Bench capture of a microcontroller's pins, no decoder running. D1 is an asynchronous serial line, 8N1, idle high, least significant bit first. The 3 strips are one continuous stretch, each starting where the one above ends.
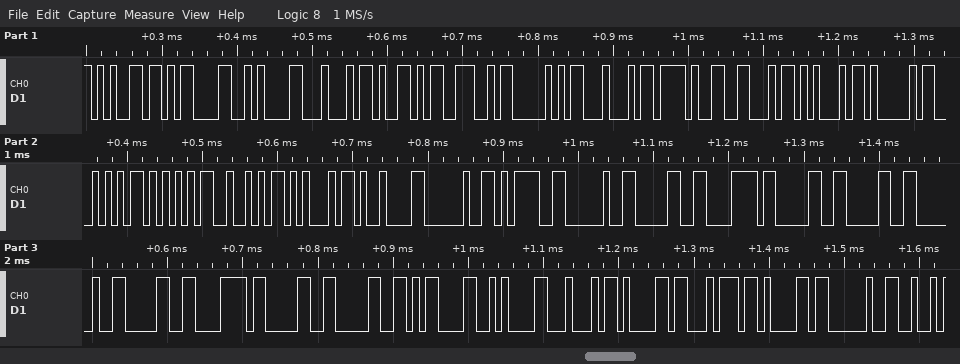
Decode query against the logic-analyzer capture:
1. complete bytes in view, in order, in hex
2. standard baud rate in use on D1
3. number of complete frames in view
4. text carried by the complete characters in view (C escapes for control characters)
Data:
65 0D 0A 44 59 4E 50 44 2F 46 45 41 54 55 52 45 09 20 3D 20 30 78 30 30 20 30 78 30 30 0D 0A 44 61 74 61 20
115200 baud
36
"e\r\nDYNPD/FEATURE\t = 0x00 0x00\r\nData "
